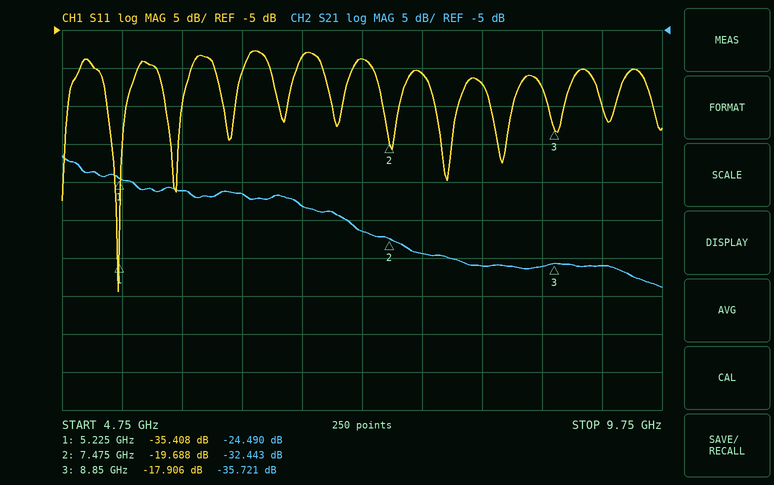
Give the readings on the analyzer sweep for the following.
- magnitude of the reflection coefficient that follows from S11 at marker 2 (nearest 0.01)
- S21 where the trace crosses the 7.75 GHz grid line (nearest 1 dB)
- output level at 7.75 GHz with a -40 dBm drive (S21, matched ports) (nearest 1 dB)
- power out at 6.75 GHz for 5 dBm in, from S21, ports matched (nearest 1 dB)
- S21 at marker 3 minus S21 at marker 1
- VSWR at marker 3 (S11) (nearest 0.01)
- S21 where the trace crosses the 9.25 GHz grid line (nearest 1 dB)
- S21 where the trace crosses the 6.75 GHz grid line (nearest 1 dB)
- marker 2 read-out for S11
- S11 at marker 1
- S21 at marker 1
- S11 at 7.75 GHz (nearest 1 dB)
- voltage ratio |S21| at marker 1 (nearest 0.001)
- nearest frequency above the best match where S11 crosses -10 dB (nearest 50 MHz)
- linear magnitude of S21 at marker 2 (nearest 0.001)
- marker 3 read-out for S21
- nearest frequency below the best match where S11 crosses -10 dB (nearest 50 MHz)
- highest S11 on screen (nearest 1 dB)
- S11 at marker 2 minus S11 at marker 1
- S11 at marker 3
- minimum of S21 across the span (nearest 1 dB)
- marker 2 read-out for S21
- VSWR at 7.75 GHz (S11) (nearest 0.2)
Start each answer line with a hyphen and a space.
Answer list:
- 0.10
- -34 dB
- -74 dBm
- -23 dBm
- -11.231 dB
- 1.29
- -36 dB
- -28 dB
- -19.688 dB
- -35.408 dB
- -24.490 dB
- -11 dB
- 0.060
- 5.40 GHz
- 0.024
- -35.721 dB
- 5.00 GHz
- -8 dB
- 15.720 dB
- -17.906 dB
- -39 dB
- -32.443 dB
- 1.8
